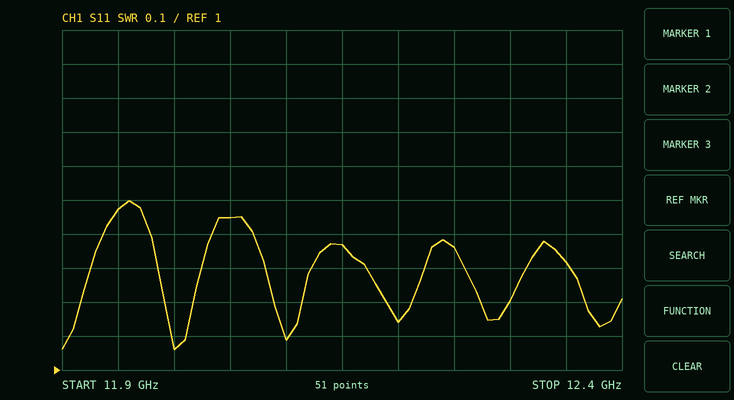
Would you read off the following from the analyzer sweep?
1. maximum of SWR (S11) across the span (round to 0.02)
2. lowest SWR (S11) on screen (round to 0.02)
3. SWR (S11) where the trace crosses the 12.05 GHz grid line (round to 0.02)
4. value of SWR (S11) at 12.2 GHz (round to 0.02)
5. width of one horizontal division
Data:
1.50
1.06
1.44
1.14
50 MHz
